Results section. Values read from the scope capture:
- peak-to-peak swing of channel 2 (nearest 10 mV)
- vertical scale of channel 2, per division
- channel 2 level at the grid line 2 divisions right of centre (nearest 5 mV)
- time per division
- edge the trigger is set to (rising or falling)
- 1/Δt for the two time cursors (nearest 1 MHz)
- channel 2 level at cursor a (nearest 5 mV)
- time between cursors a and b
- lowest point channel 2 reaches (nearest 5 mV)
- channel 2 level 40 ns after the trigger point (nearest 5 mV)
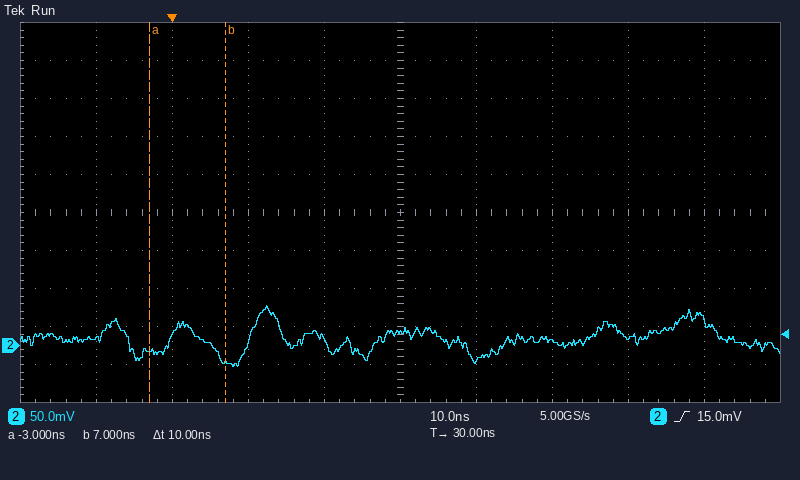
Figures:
80 mV
50 mV
5 mV
10 ns
rising
100 MHz
-5 mV
10 ns
-30 mV
-20 mV
